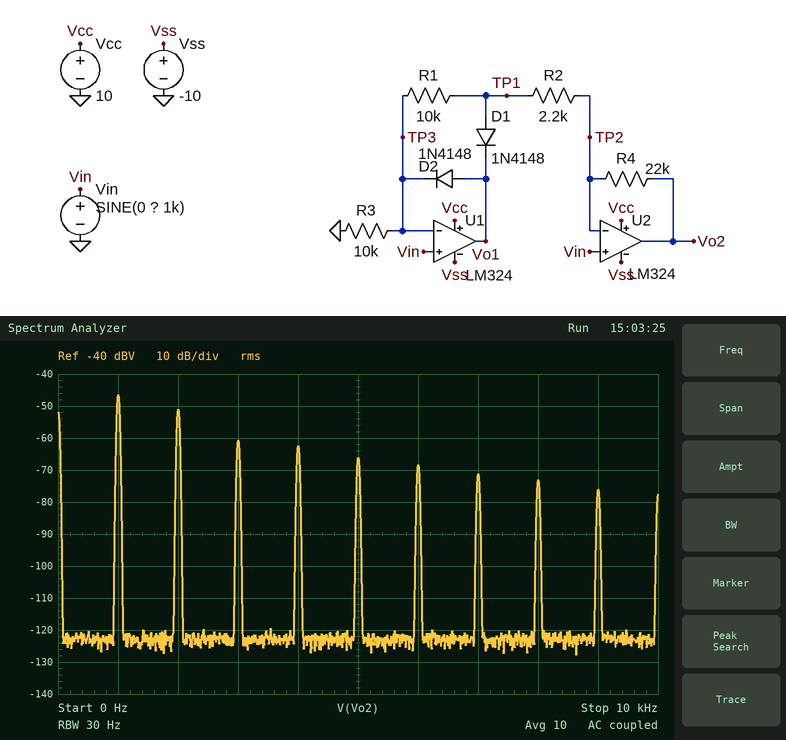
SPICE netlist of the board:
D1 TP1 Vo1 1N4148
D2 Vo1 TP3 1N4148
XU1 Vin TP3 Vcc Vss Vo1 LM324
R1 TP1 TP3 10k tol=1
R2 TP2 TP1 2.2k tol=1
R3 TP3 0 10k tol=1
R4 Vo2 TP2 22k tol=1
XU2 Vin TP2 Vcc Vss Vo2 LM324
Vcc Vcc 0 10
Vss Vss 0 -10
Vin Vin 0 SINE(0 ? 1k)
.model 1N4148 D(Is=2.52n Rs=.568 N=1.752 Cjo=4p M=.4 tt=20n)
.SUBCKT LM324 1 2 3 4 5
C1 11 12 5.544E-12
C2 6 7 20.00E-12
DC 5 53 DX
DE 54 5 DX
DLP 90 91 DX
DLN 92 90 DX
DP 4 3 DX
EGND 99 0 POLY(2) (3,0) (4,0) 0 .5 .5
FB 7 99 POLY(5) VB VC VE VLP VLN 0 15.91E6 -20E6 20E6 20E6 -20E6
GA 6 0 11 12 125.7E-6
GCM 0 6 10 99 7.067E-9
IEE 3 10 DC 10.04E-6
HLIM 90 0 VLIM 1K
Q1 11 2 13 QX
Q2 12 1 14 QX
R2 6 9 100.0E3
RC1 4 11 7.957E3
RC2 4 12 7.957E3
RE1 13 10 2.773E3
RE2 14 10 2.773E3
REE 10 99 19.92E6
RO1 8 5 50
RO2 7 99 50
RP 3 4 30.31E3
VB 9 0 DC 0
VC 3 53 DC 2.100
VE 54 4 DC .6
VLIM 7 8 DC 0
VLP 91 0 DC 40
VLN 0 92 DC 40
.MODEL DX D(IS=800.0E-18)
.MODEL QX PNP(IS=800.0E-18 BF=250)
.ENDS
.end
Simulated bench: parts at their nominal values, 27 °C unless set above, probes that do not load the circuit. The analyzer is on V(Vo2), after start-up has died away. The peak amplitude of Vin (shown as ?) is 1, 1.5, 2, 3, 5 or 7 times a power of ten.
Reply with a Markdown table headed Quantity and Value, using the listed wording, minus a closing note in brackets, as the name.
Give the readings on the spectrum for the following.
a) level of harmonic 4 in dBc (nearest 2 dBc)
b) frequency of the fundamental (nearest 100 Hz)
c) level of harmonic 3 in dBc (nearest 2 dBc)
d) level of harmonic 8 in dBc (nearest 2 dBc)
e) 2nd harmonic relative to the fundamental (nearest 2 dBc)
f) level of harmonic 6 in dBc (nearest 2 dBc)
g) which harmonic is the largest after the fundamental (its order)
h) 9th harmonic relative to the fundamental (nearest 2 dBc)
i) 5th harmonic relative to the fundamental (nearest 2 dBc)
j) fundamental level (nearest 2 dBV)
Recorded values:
| Quantity | Value |
|---|---|
| level of harmonic 4 in dBc | -16 dBc |
| frequency of the fundamental | 1.0 kHz |
| level of harmonic 3 in dBc | -14 dBc |
| level of harmonic 8 in dBc | -26 dBc |
| 2nd harmonic relative to the fundamental | -4 dBc |
| level of harmonic 6 in dBc | -22 dBc |
| which harmonic is the largest after the fundamental | 2 |
| 9th harmonic relative to the fundamental | -30 dBc |
| 5th harmonic relative to the fundamental | -20 dBc |
| fundamental level | -46 dBV |
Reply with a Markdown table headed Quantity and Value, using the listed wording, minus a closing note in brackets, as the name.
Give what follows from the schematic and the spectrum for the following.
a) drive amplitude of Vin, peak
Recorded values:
| Quantity | Value |
|---|---|
| drive amplitude of Vin, peak | 1.5 mV |
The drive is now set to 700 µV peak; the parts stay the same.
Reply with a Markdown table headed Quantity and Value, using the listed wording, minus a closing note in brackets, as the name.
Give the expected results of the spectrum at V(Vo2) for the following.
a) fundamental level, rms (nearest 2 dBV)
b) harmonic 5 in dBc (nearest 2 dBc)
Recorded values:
| Quantity | Value |
|---|---|
| fundamental level, rms | -52 dBV |
| harmonic 5 in dBc | -22 dBc |
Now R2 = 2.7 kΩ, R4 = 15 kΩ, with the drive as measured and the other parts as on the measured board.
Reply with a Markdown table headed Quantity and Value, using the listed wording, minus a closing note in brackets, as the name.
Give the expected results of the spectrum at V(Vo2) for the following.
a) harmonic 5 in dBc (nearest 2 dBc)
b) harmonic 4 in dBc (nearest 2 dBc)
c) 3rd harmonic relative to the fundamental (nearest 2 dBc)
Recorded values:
| Quantity | Value |
|---|---|
| harmonic 5 in dBc | -18 dBc |
| harmonic 4 in dBc | -14 dBc |
| 3rd harmonic relative to the fundamental | -12 dBc |
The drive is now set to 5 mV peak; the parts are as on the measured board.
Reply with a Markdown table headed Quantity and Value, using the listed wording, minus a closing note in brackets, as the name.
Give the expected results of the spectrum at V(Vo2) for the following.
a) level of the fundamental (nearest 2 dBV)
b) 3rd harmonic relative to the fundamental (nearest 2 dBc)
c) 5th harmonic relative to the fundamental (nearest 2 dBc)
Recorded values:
| Quantity | Value |
|---|---|
| level of the fundamental | -36 dBV |
| 3rd harmonic relative to the fundamental | -18 dBc |
| 5th harmonic relative to the fundamental | -22 dBc |
